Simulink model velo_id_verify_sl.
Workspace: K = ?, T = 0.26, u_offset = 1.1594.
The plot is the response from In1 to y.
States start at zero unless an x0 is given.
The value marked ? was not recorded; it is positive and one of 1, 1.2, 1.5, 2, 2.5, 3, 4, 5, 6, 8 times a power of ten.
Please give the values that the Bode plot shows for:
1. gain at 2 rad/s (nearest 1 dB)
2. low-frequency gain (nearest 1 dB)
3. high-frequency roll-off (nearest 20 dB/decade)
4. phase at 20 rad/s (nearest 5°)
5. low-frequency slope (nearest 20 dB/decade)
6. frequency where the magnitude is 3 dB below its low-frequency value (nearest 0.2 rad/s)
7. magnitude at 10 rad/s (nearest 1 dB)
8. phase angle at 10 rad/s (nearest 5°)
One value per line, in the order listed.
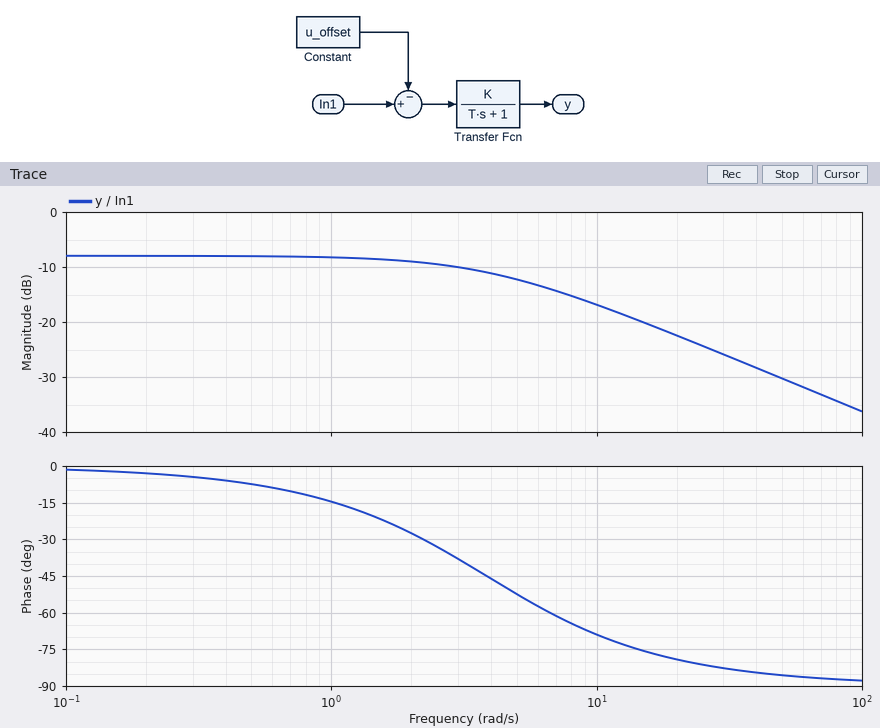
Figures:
-9 dB
-8 dB
-20 dB/decade
-80°
0 dB/decade
3.8 rad/s
-17 dB
-70°
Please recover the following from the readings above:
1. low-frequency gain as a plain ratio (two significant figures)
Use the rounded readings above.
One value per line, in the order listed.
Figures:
0.40
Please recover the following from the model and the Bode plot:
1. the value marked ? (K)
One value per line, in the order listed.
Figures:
0.4
